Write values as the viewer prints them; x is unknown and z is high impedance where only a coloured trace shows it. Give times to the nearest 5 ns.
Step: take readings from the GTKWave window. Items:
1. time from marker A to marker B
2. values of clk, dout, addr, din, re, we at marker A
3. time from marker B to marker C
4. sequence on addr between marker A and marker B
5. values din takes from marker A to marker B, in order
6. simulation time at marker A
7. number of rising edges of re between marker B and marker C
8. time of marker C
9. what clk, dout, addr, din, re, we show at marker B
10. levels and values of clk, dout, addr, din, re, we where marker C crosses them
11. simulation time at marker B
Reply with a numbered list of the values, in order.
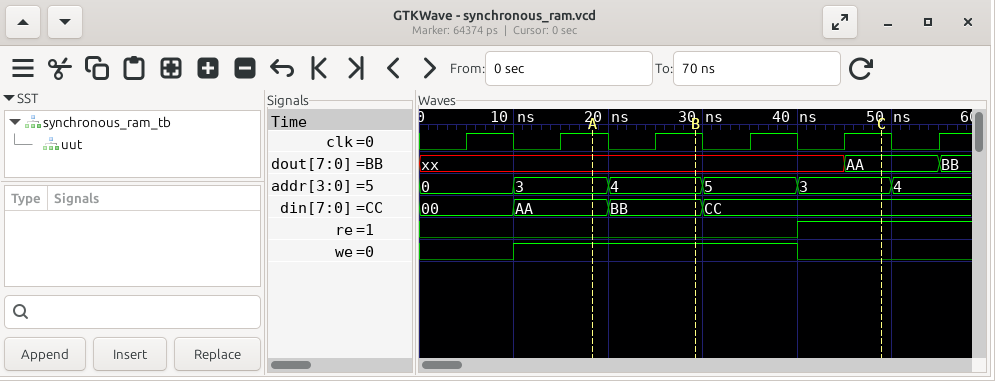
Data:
1. 10 ns
2. clk=1, dout=xx, addr=3, din=AA, re=0, we=1
3. 20 ns
4. 3, 4
5. AA, BB
6. 20 ns
7. 1
8. 50 ns
9. clk=1, dout=xx, addr=4, din=BB, re=0, we=1
10. clk=1, dout=AA, addr=3, din=CC, re=1, we=0
11. 30 ns
